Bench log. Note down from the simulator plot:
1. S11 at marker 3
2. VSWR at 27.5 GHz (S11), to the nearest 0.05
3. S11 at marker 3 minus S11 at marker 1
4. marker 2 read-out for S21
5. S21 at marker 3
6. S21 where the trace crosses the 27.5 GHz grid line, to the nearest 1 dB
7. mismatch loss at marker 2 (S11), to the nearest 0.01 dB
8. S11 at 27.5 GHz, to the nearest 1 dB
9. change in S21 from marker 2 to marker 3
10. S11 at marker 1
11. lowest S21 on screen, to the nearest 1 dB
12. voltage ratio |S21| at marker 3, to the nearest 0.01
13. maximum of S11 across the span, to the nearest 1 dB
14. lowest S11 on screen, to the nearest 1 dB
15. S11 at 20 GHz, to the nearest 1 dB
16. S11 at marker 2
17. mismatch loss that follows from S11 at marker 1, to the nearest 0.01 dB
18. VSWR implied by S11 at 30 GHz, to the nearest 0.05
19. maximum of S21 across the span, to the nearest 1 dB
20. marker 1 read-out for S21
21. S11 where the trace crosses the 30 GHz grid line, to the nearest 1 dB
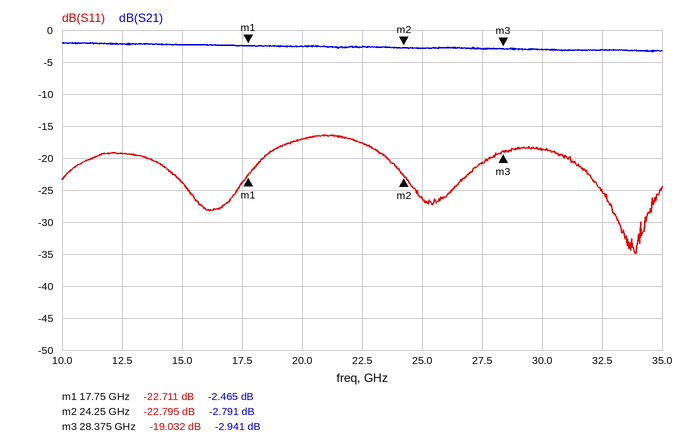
-19.032 dB
1.20
3.679 dB
-2.791 dB
-2.941 dB
-3 dB
0.02 dB
-21 dB
-0.150 dB
-22.711 dB
-3 dB
0.71
-16 dB
-35 dB
-17 dB
-22.795 dB
0.02 dB
1.25
-2 dB
-2.465 dB
-19 dB
